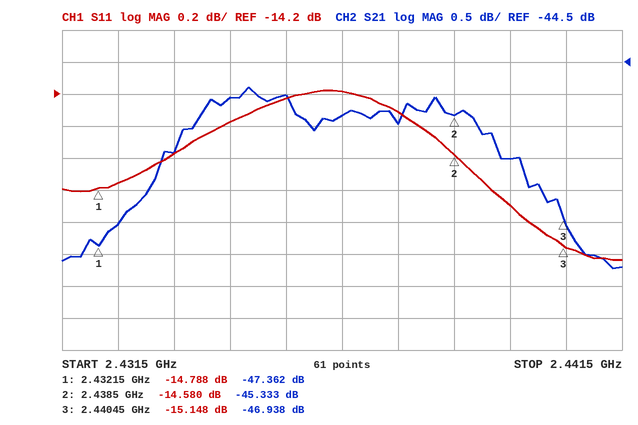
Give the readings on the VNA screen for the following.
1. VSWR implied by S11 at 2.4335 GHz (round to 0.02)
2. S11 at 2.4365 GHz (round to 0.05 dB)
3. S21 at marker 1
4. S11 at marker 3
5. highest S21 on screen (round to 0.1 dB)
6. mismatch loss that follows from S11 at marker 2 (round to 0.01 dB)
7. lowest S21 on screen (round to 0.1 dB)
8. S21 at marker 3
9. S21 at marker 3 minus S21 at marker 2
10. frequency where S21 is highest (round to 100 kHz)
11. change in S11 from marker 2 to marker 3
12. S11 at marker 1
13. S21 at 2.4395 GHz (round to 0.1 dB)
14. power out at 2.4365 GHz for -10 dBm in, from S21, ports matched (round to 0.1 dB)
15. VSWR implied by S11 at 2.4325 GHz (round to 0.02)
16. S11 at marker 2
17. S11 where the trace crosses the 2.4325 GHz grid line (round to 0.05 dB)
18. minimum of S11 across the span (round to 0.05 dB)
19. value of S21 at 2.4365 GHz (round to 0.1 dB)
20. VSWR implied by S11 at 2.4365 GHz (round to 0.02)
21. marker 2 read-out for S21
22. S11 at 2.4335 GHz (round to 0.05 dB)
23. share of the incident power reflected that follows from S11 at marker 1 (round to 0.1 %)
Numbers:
1.46
-14.20 dB
-47.362 dB
-15.148 dB
-44.9 dB
0.15 dB
-47.7 dB
-46.938 dB
-1.605 dB
2.4348 GHz
-0.568 dB
-14.788 dB
-46.0 dB
-55.3 dBm
1.44
-14.580 dB
-14.75 dB
-15.25 dB
-45.3 dB
1.48
-45.333 dB
-14.55 dB
3.3 %
